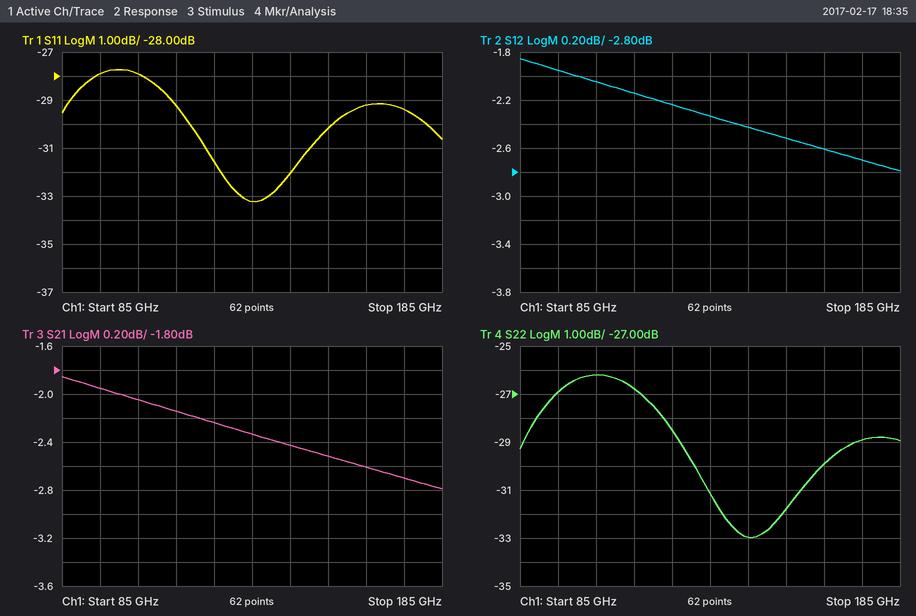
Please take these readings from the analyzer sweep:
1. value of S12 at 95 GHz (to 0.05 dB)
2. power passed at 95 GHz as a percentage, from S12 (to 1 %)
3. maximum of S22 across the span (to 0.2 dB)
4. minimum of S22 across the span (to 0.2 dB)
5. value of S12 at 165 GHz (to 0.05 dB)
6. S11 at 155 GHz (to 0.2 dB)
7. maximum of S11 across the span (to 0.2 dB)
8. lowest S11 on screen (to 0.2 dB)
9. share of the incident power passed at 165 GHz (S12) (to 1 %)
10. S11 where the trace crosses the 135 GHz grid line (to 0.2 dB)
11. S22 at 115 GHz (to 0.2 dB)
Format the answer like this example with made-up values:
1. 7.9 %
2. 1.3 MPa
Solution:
1. -1.95 dB
2. 64 %
3. -26.2 dB
4. -33.0 dB
5. -2.60 dB
6. -30.2 dB
7. -27.8 dB
8. -33.2 dB
9. 55 %
10. -33.2 dB
11. -26.8 dB
